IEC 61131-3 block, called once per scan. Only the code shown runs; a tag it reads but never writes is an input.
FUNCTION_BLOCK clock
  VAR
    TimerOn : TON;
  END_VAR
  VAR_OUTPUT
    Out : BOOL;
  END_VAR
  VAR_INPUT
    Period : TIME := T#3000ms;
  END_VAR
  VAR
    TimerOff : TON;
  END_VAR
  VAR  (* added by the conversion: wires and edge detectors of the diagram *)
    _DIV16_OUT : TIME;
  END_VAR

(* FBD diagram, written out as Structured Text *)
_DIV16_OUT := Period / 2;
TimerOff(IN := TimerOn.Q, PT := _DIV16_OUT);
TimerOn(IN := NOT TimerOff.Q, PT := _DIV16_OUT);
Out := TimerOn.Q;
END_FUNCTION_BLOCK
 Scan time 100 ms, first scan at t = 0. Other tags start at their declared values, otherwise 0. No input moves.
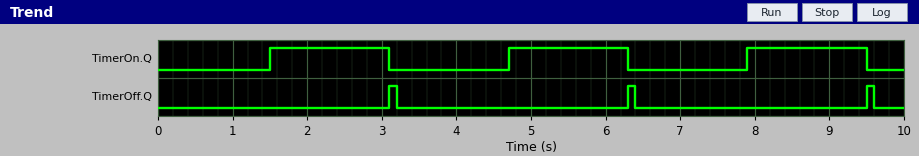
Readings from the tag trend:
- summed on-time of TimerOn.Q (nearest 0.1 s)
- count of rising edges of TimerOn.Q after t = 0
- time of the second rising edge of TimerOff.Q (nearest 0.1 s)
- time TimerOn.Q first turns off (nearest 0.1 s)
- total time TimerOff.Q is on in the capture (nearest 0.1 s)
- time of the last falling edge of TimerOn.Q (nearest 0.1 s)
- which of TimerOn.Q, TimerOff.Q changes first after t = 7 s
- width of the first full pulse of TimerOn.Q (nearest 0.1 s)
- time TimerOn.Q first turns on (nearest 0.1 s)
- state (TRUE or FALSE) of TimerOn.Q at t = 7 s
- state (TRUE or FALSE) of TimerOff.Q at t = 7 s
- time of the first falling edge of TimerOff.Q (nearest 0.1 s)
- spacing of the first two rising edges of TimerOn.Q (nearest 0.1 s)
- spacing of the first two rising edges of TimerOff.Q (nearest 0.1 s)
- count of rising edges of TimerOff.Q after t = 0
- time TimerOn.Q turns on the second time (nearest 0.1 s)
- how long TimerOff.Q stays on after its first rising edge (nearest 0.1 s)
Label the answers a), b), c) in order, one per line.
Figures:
a) 4.8 s
b) 3
c) 6.3 s
d) 3.1 s
e) 0.3 s
f) 9.5 s
g) TimerOn.Q
h) 1.6 s
i) 1.5 s
j) FALSE
k) FALSE
l) 3.2 s
m) 3.2 s
n) 3.2 s
o) 3
p) 4.7 s
q) 0.1 s
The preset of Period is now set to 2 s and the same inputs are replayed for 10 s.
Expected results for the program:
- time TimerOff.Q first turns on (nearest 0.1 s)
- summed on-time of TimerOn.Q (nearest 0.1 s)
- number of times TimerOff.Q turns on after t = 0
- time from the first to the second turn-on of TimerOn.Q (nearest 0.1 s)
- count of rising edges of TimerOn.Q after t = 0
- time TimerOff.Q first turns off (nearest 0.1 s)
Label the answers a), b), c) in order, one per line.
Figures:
a) 2.1 s
b) 4.6 s
c) 4
d) 2.2 s
e) 5
f) 2.2 s
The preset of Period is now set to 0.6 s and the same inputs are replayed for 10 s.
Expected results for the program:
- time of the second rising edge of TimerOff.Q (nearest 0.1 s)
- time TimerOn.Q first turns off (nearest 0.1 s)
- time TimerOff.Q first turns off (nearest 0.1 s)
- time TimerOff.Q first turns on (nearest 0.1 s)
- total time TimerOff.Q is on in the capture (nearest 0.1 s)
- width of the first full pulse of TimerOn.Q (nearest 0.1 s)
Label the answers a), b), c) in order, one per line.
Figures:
a) 1.5 s
b) 0.7 s
c) 0.8 s
d) 0.7 s
e) 1.2 s
f) 0.4 s
